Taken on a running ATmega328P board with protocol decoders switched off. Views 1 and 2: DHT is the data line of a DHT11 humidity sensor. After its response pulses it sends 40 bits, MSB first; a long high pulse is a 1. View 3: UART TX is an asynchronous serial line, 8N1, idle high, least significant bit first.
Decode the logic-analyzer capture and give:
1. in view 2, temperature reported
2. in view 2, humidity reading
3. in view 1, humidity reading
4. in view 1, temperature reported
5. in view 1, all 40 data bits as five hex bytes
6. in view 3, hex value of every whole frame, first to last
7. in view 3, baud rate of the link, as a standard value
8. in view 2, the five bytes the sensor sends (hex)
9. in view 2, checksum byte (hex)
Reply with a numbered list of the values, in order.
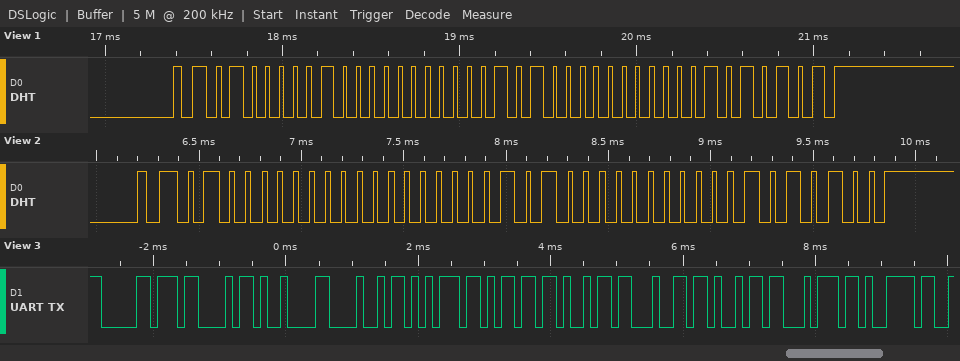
1. 20.0 °C
2. 64 %
3. 65 %
4. 20.0 °C
5. 41 00 14 00 55
6. B0 43 09 48 75 6D 69 64 69 74 79
7. 9600 baud
8. 40 00 14 00 54
9. 0x54
